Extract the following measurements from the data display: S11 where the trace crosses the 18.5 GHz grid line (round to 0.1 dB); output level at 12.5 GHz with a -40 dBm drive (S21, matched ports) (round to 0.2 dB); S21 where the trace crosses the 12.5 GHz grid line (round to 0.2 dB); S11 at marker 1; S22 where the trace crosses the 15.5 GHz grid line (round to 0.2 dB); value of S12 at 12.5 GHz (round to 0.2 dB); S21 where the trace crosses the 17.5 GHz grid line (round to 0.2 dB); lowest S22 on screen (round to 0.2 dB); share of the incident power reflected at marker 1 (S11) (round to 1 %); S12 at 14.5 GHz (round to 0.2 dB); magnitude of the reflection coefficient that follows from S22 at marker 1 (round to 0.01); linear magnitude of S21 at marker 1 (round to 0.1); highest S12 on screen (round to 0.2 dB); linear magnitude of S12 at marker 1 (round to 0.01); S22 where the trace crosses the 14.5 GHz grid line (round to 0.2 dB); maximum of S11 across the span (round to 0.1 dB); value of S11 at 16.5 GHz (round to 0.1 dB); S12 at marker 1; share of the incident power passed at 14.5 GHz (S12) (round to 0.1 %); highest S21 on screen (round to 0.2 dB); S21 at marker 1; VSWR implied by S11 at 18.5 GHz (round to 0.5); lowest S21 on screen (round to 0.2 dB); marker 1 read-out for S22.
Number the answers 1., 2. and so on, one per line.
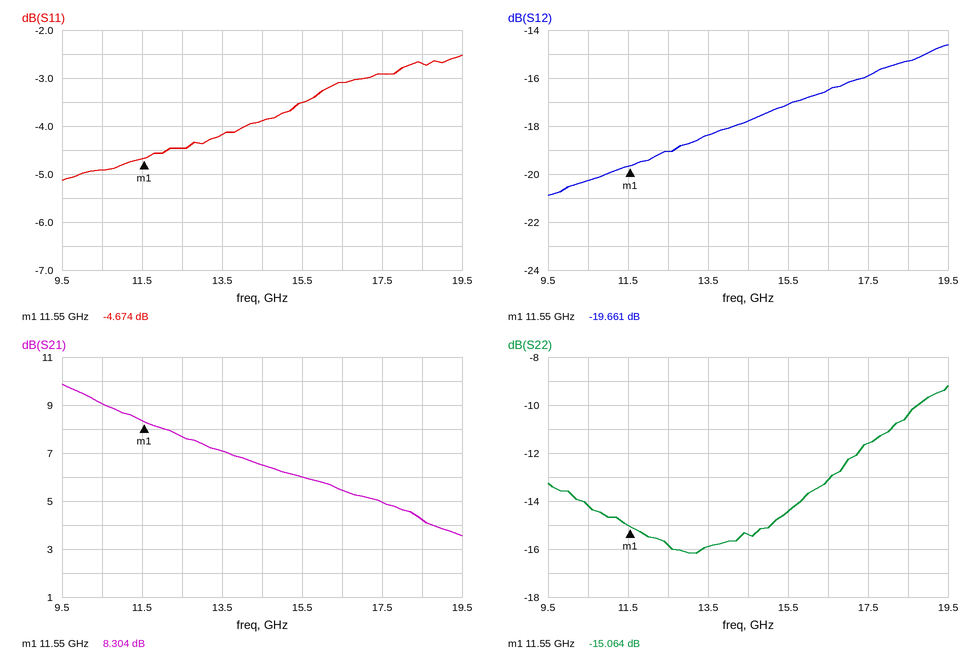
1. -2.7 dB
2. -32.4 dBm
3. 7.6 dB
4. -4.674 dB
5. -14.4 dB
6. -19.0 dB
7. 5.0 dB
8. -16.2 dB
9. 34 %
10. -17.8 dB
11. 0.18
12. 2.6
13. -14.6 dB
14. 0.10
15. -15.4 dB
16. -2.5 dB
17. -3.1 dB
18. -19.661 dB
19. 1.7 %
20. 9.8 dB
21. 8.304 dB
22. 6.5
23. 3.6 dB
24. -15.064 dB
